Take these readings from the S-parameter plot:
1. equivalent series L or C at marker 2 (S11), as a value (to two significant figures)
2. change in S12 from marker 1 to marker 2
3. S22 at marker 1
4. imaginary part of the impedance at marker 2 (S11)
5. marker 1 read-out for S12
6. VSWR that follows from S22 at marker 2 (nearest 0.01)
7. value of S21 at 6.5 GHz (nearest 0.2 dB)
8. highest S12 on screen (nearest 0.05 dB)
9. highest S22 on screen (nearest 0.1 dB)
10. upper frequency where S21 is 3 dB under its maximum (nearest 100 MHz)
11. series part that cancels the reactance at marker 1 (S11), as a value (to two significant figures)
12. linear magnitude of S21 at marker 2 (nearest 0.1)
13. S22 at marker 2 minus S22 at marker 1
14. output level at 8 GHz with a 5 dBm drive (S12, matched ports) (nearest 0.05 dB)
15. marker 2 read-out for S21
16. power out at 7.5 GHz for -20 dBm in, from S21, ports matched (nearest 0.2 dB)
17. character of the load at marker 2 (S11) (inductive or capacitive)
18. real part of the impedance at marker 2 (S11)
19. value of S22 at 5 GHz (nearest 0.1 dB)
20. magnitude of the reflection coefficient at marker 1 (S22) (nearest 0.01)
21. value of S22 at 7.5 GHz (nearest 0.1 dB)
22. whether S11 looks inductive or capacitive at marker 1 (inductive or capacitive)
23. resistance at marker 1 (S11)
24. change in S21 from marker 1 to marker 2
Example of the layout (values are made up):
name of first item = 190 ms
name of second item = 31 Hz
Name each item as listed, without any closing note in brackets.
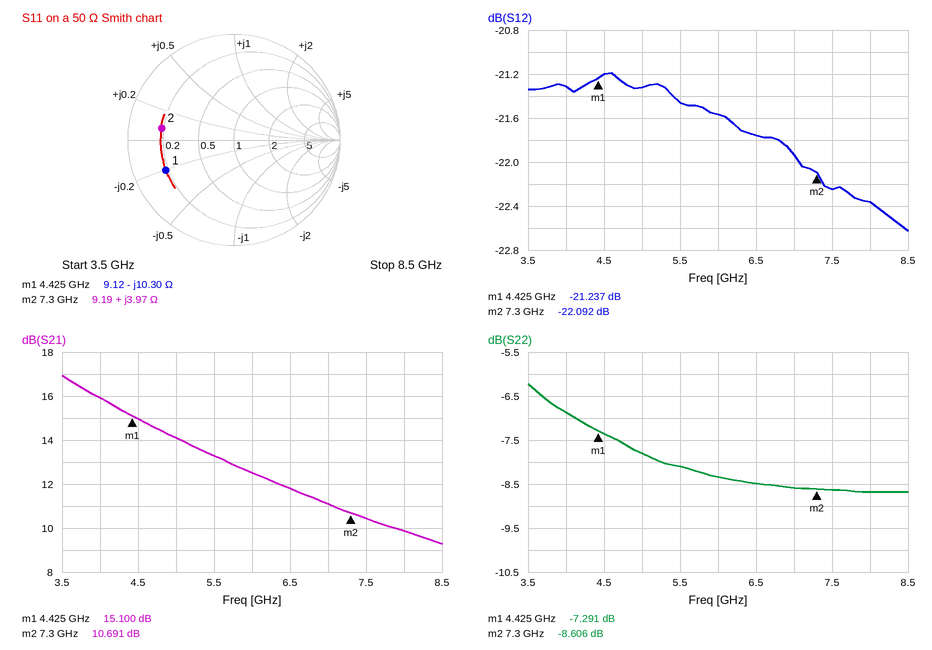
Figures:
equivalent series L or C at marker 2 (S11), as a value = 87 pH
change in S12 from marker 1 to marker 2 = -0.855 dB
S22 at marker 1 = -7.291 dB
imaginary part of the impedance at marker 2 = +3.97 Ω
marker 1 read-out for S12 = -21.237 dB
VSWR that follows from S22 at marker 2 = 2.18
value of S21 at 6.5 GHz = 11.8 dB
highest S12 on screen = -21.20 dB
highest S22 on screen = -6.2 dB
upper frequency where S21 is 3 dB under its maximum = 5.1 GHz
series part that cancels the reactance at marker 1 (S11), as a value = 370 pH
linear magnitude of S21 at marker 2 = 3.4
S22 at marker 2 minus S22 at marker 1 = -1.315 dB
output level at 8 GHz with a 5 dBm drive (S12, matched ports) = -17.35 dBm
marker 2 read-out for S21 = 10.691 dB
power out at 7.5 GHz for -20 dBm in, from S21, ports matched = -9.6 dBm
character of the load at marker 2 (S11) = inductive
real part of the impedance at marker 2 = 9.19 Ω
value of S22 at 5 GHz = -7.8 dB
magnitude of the reflection coefficient at marker 1 (S22) = 0.43
value of S22 at 7.5 GHz = -8.6 dB
whether S11 looks inductive or capacitive at marker 1 = capacitive
resistance at marker 1 = 9.12 Ω
change in S21 from marker 1 to marker 2 = -4.409 dB
